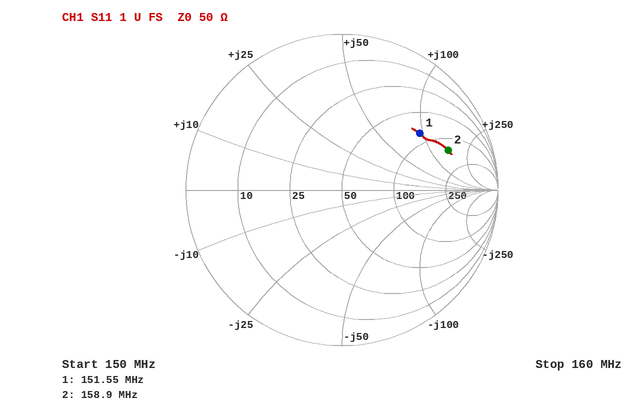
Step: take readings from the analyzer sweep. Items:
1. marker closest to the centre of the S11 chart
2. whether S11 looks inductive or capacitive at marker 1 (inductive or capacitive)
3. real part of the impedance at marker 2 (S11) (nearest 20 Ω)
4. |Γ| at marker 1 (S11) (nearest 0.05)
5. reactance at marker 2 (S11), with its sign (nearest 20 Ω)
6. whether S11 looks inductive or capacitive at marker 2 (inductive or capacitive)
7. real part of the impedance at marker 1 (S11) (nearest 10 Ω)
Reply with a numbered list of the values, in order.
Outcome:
1. marker 1
2. inductive
3. 140 Ω
4. 0.60
5. +160 Ω
6. inductive
7. 80 Ω
